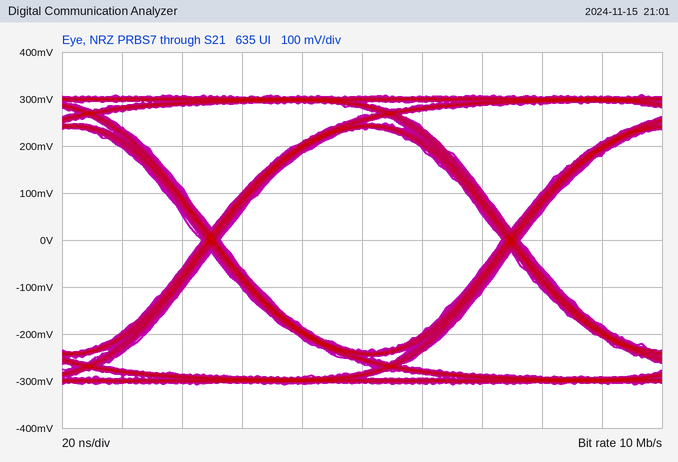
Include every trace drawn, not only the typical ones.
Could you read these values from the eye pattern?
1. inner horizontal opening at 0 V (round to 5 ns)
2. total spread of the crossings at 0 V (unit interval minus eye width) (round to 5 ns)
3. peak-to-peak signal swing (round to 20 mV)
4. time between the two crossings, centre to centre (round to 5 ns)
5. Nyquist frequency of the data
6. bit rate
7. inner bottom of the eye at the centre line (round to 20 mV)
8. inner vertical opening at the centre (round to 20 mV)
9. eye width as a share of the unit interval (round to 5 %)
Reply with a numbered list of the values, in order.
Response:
1. 95 ns
2. 5 ns
3. 620 mV
4. 100 ns
5. 5 MHz
6. 10 Mb/s
7. -240 mV
8. 480 mV
9. 95 %
